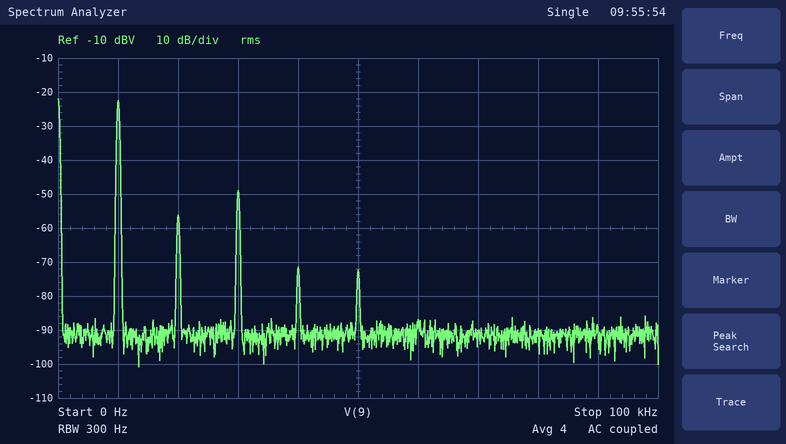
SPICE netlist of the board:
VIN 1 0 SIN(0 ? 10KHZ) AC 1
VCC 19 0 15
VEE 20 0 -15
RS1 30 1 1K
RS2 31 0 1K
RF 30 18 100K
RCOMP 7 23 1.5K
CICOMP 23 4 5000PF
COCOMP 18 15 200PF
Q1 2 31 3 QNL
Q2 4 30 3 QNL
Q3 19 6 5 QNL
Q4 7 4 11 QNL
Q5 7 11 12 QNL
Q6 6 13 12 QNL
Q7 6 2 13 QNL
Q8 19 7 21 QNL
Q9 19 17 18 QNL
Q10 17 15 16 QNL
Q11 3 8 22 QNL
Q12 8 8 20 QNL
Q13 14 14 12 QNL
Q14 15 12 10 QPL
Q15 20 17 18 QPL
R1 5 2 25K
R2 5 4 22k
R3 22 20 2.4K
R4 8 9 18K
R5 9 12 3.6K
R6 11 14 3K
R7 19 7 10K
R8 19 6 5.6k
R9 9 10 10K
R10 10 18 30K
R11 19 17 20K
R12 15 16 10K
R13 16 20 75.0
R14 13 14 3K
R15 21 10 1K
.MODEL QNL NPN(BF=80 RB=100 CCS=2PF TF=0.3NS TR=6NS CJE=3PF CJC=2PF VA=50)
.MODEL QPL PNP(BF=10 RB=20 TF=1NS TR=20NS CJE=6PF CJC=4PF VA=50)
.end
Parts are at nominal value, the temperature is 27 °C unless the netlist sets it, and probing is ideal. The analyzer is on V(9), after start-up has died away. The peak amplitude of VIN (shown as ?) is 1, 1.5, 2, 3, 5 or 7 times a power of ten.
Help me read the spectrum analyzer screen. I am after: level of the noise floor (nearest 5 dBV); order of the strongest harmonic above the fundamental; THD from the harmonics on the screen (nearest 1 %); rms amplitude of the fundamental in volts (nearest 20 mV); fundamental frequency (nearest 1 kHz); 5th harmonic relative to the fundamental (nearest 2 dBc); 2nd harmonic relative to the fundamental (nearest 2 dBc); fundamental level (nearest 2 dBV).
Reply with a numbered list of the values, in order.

1. -90 dBV
2. 3
3. 5 %
4. 80 mV
5. 10 kHz
6. -50 dBc
7. -34 dBc
8. -22 dBV
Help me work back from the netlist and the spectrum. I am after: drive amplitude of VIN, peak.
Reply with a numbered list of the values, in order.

1. 50 mV
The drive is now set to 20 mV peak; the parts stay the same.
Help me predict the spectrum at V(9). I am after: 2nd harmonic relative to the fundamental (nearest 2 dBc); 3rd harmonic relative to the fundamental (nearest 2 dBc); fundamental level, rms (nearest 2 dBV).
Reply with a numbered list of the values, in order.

1. -42 dBc
2. -42 dBc
3. -30 dBV
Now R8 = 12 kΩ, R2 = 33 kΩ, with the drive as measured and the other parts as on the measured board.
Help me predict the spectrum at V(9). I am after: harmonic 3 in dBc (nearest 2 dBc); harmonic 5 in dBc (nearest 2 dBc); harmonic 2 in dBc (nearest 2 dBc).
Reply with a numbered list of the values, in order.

1. -32 dBc
2. -58 dBc
3. -24 dBc
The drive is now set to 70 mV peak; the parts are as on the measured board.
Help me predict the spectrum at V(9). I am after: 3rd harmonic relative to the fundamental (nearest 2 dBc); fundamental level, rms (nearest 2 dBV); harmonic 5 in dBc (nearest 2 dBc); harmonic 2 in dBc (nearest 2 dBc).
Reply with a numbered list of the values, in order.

1. -22 dBc
2. -20 dBV
3. -40 dBc
4. -30 dBc
